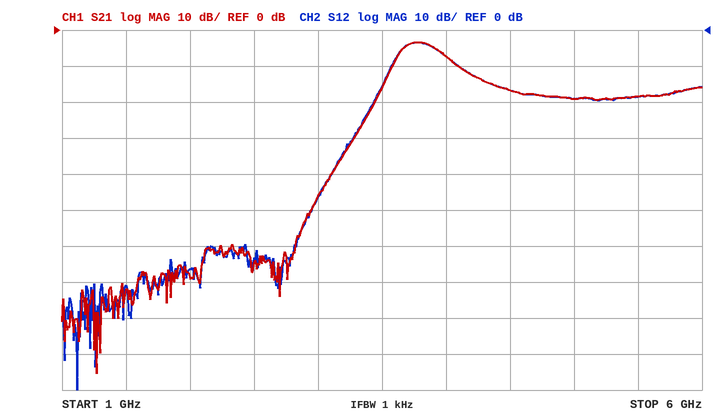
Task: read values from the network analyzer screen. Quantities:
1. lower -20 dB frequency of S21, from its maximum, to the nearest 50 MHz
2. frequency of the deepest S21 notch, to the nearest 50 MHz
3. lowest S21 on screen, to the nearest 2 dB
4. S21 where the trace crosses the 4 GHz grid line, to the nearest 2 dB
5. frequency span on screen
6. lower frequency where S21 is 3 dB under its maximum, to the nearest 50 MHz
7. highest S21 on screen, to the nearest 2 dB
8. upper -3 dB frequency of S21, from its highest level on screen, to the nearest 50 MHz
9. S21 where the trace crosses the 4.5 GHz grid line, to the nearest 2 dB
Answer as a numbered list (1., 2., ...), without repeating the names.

1. 3.40 GHz
2. 1.25 GHz
3. -96 dB
4. -8 dB
5. 5 GHz
6. 3.65 GHz
7. -4 dB
8. 3.95 GHz
9. -16 dB
